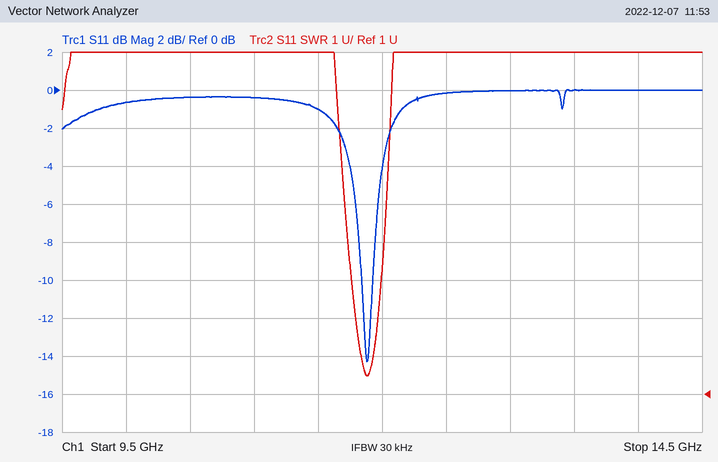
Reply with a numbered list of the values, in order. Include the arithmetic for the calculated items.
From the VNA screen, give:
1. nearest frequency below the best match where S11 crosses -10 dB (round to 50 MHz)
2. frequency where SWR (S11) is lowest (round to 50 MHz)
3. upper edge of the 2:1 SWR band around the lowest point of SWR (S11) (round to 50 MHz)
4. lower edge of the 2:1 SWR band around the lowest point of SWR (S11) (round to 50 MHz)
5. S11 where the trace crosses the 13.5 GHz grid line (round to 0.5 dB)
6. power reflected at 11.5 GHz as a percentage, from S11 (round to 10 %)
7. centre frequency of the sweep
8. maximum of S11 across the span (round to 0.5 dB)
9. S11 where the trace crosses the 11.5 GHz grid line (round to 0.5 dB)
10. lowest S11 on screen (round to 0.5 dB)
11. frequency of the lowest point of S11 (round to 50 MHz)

1. 11.85 GHz
2. 11.90 GHz
3. 11.95 GHz
4. 11.85 GHz
5. 0.0 dB
6. 10^(-1/10) ≈ 79.4 %, so 80 % to the nearest 10 %
7. 12 GHz
8. 0.0 dB
9. -1.0 dB
10. -14.5 dB
11. 11.90 GHz
